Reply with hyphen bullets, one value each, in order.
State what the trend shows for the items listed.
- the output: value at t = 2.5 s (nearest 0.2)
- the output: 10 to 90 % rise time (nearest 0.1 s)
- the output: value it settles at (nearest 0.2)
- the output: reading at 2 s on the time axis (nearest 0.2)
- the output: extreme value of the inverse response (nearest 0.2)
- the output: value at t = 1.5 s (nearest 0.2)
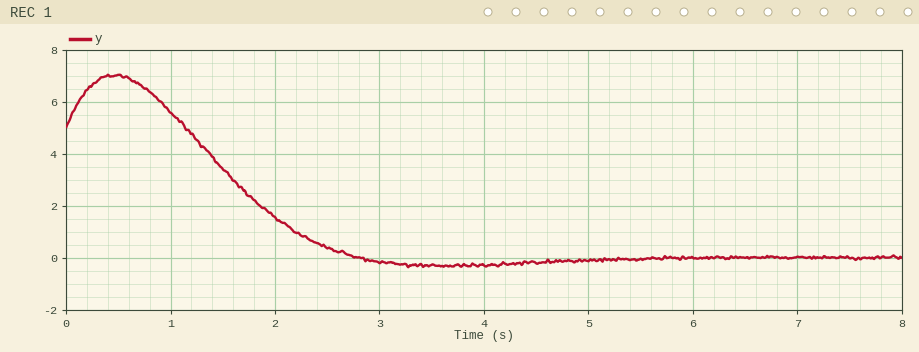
- 0.4
- 1.2 s
- 0.0
- 1.6
- 7.0
- 3.4
